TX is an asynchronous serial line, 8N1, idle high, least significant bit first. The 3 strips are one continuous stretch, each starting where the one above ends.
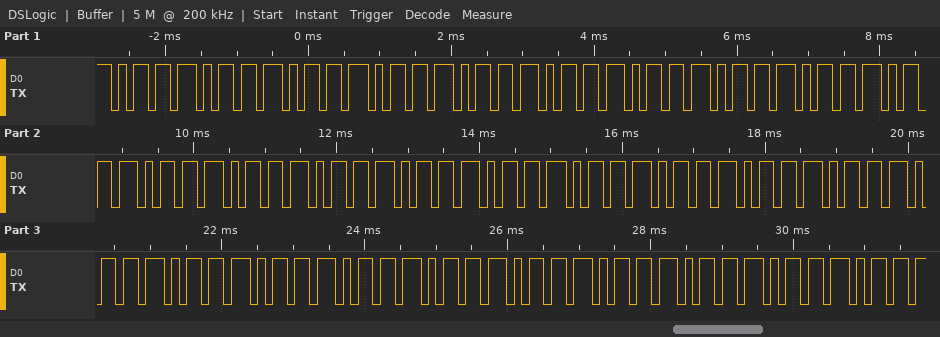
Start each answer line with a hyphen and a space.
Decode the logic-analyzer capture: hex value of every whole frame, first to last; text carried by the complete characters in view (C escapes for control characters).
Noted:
- 6D 6D 6D 6D 6D 6D 6D 6D 6D 6D 6D 6D 6D 6D 6D 6D 6D 6D 6D 6D 6D 6D 6D 6D 6D 6D 6D 6D 6D
- "mmmmmmmmmmmmmmmmmmmmmmmmmmmmm"
